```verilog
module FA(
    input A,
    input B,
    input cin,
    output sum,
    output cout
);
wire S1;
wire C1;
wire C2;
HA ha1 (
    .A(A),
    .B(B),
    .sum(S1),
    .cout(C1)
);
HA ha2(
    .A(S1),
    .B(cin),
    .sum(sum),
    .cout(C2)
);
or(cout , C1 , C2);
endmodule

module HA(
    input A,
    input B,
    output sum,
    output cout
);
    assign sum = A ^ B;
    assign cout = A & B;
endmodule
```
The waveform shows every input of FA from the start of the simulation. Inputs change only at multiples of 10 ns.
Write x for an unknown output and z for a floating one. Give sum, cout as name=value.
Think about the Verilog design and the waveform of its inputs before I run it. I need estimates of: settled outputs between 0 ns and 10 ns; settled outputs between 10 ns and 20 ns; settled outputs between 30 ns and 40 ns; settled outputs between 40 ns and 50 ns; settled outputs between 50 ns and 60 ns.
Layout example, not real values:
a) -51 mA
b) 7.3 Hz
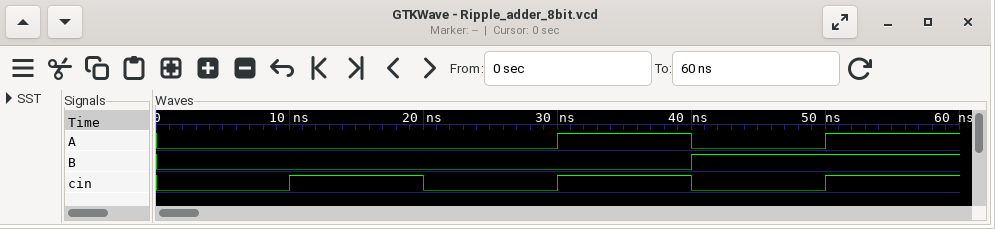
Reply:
a) sum=0, cout=0
b) sum=1, cout=0
c) sum=0, cout=1
d) sum=1, cout=0
e) sum=1, cout=1
